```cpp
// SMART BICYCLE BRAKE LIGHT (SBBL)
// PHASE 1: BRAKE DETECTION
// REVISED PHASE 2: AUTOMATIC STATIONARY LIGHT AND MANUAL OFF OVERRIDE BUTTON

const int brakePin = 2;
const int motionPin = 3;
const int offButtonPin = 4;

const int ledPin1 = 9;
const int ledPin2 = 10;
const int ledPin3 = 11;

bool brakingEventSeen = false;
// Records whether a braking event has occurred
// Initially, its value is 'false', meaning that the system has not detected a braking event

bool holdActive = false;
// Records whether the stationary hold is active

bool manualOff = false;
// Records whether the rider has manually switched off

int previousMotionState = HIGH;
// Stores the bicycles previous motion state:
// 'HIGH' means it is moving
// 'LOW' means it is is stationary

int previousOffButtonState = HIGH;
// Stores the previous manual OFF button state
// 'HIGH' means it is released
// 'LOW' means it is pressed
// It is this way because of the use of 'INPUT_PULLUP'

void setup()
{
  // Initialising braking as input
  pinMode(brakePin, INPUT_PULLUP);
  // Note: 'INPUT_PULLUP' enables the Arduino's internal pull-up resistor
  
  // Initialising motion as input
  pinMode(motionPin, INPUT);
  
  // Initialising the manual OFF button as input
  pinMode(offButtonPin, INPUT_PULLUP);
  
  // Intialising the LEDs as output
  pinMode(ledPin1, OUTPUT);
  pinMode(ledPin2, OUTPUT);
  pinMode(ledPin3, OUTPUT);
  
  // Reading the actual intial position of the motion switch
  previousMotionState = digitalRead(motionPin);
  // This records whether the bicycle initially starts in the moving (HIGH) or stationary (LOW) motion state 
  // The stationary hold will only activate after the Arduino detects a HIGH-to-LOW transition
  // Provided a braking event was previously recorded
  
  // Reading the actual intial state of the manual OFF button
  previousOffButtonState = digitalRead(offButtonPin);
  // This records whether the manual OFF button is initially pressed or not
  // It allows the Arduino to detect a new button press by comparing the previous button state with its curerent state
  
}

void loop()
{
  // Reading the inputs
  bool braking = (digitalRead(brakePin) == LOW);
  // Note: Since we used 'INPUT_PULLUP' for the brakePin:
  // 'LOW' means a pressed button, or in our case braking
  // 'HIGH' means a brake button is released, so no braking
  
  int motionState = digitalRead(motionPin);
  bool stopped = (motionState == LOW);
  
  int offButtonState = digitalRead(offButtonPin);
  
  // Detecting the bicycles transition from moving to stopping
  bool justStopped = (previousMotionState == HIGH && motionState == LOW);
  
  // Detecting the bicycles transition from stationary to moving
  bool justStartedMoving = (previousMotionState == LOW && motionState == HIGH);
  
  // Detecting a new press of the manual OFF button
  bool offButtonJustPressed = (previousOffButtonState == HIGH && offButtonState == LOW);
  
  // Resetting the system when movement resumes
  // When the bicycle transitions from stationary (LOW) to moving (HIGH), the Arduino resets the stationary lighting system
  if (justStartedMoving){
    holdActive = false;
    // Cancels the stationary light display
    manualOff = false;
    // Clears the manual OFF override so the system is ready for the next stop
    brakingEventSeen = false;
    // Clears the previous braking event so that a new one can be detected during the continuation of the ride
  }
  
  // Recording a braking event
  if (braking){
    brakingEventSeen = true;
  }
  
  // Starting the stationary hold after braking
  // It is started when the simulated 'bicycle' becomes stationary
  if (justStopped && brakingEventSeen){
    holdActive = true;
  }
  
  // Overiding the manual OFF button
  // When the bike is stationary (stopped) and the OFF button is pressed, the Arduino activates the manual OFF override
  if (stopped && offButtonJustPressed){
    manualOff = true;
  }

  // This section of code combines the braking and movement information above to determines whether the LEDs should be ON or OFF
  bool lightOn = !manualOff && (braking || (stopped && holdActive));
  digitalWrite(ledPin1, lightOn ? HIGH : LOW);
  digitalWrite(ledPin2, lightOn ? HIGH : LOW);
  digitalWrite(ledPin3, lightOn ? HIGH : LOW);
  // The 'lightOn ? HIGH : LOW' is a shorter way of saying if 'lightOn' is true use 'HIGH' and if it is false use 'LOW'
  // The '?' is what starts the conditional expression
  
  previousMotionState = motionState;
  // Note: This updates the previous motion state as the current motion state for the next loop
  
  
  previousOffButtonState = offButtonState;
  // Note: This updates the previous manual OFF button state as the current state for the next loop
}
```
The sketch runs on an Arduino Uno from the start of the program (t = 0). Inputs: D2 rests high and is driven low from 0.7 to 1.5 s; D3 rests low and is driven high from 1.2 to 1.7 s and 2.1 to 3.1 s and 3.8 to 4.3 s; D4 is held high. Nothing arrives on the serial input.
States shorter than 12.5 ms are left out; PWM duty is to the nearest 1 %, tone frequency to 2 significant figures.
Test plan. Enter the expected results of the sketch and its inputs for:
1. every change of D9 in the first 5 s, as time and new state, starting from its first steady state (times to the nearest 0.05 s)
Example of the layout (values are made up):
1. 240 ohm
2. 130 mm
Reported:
1. 0 s low; 0.7 s high; 1.5 s low; 1.7 s high; 2.1 s low
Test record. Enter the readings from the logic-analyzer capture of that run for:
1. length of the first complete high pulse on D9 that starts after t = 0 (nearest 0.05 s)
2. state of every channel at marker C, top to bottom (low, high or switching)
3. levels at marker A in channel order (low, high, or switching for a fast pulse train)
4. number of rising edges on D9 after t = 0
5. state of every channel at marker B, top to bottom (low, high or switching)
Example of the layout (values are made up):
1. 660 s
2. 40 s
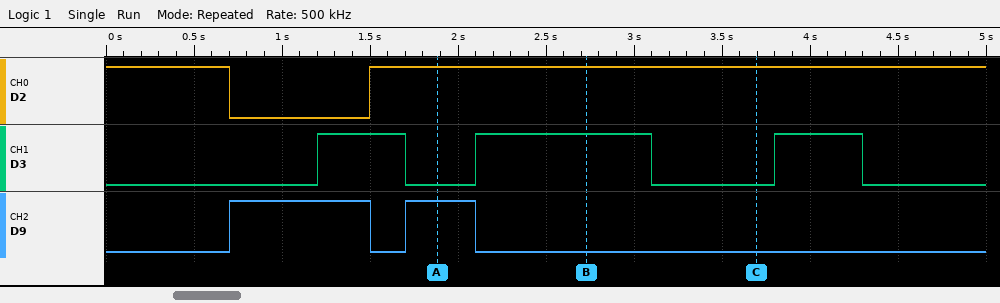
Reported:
1. 0.80 s
2. D2 high, D3 low, D9 low
3. D2 high, D3 low, D9 high
4. 2
5. D2 high, D3 high, D9 low
